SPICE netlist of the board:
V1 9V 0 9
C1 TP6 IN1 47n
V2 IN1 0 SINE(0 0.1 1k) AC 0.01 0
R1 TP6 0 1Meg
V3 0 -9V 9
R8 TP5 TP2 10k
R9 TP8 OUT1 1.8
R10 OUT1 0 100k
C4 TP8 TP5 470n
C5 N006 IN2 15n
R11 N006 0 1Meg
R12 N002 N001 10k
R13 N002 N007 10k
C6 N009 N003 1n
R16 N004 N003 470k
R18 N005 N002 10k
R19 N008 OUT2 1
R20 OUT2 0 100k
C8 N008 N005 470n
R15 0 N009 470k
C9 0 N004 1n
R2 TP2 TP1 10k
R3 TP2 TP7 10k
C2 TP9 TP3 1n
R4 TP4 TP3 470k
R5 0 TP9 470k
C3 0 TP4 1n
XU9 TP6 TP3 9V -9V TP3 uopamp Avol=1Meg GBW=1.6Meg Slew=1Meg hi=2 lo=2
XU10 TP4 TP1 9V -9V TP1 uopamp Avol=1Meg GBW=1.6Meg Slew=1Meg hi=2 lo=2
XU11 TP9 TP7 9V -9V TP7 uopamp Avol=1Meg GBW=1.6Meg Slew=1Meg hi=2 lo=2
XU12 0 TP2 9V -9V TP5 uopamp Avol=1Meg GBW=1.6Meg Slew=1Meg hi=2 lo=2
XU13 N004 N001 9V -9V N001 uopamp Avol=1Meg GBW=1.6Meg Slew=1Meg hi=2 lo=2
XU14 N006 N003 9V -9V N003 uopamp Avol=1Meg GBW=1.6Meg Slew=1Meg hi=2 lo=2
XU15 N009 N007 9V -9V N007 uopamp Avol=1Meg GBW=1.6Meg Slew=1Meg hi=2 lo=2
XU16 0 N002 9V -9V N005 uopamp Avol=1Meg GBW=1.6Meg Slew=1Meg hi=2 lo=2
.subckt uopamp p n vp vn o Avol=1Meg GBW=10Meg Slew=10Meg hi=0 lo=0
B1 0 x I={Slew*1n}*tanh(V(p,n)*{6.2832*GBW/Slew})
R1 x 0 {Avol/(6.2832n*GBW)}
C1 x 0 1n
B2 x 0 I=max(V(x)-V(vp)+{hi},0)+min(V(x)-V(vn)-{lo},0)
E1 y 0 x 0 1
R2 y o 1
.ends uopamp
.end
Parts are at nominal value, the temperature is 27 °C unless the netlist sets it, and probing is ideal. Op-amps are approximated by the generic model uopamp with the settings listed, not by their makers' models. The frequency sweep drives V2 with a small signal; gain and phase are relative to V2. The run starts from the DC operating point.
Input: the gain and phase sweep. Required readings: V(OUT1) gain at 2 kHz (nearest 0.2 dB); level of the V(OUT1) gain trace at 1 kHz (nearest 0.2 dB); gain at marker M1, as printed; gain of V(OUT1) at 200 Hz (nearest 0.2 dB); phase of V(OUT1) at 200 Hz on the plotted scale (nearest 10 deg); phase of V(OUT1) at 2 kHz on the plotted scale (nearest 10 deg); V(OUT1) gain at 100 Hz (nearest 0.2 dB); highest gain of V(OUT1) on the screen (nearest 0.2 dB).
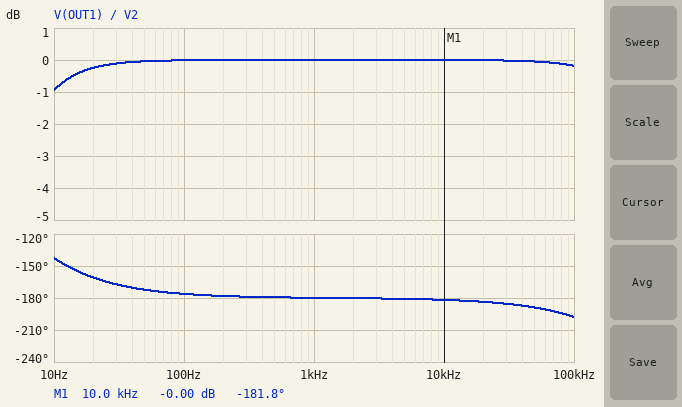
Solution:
0 dB
0 dB
-0.00 dB
0 dB
-180 deg
-180 deg
0 dB
0 dB
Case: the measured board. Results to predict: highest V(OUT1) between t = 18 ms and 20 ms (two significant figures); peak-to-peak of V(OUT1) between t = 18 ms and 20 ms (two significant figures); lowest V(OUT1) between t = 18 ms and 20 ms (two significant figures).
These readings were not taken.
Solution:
100 mV
200 mV
-100 mV
